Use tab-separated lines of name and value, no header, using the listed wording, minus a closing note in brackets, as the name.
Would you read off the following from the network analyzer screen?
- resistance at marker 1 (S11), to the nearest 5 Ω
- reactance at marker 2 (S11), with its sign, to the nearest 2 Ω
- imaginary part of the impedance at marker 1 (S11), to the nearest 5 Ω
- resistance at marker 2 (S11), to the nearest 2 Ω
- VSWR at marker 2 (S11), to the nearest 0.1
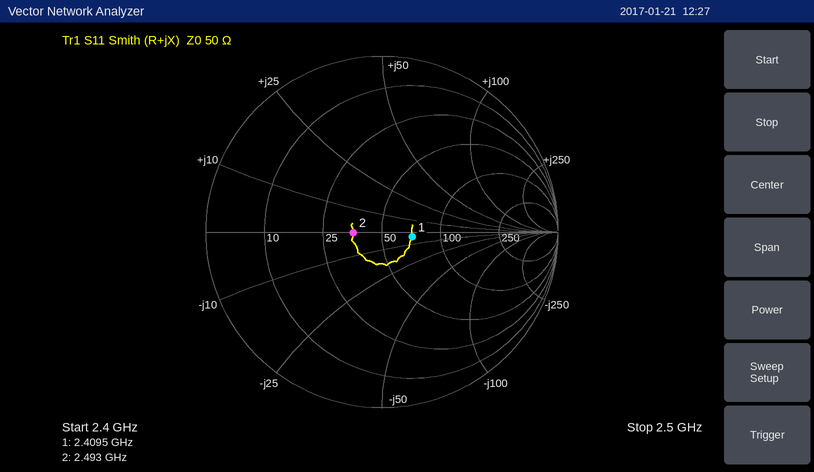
resistance at marker 1 (S11), to the nearest 5 Ω	70 Ω
reactance at marker 2 (S11), with its sign, to the nearest 2 Ω	0 Ω
imaginary part of the impedance at marker 1 (S11), to the nearest 5 Ω	-5 Ω
resistance at marker 2 (S11), to the nearest 2 Ω	36 Ω
VSWR at marker 2 (S11), to the nearest 0.1	1.4
